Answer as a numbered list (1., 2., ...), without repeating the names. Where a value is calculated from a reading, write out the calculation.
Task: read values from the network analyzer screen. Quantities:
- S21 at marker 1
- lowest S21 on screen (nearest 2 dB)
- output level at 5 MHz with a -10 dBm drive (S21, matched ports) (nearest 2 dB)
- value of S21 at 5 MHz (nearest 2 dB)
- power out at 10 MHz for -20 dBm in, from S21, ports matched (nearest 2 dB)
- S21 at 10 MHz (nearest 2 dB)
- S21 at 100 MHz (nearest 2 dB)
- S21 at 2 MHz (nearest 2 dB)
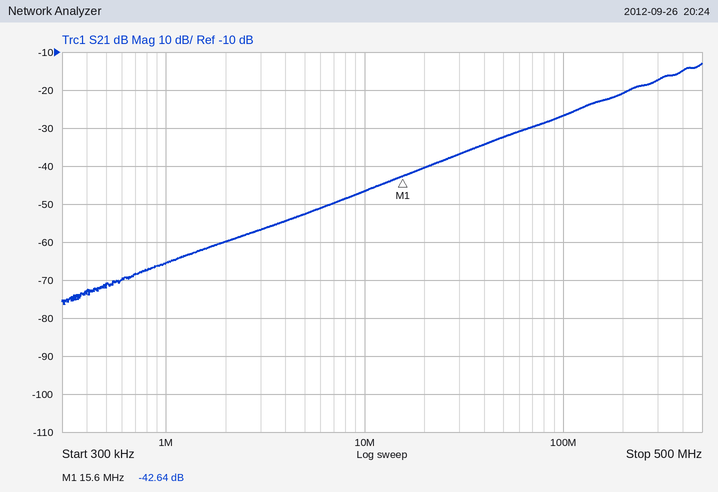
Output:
1. -42.64 dB
2. -76 dB
3. -10 dBm + (-52 dB) = -62 dBm
4. -52 dB
5. -20 dBm + (-46 dB) = -66 dBm
6. -46 dB
7. -26 dB
8. -60 dB
